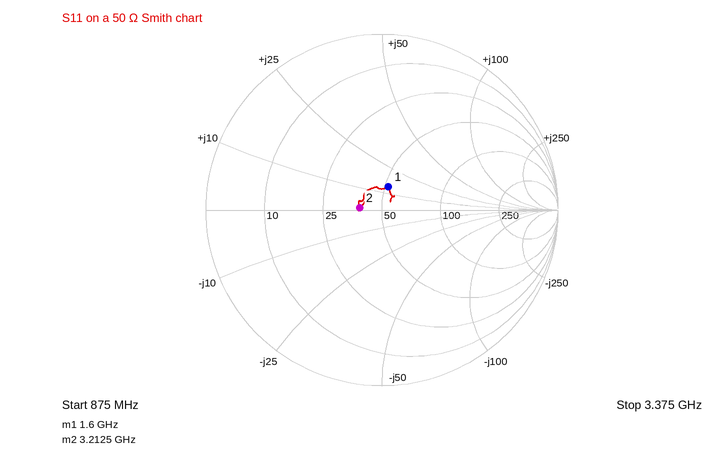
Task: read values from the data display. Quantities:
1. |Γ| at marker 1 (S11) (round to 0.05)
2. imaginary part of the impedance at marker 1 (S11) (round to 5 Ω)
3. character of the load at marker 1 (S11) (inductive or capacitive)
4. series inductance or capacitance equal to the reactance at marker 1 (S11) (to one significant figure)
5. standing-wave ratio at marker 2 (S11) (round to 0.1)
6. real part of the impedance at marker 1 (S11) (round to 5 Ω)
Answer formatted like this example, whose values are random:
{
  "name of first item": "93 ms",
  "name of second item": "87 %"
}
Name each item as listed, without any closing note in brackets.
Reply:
{
  "|Γ| at marker 1 (S11)": "0.15",
  "imaginary part of the impedance at marker 1 (S11)": "+15 Ω",
  "character of the load at marker 1 (S11)": "inductive",
  "series inductance or capacitance equal to the reactance at marker 1 (S11)": "1 nH",
  "standing-wave ratio at marker 2 (S11)": "1.3",
  "real part of the impedance at marker 1 (S11)": "50 Ω"
}
